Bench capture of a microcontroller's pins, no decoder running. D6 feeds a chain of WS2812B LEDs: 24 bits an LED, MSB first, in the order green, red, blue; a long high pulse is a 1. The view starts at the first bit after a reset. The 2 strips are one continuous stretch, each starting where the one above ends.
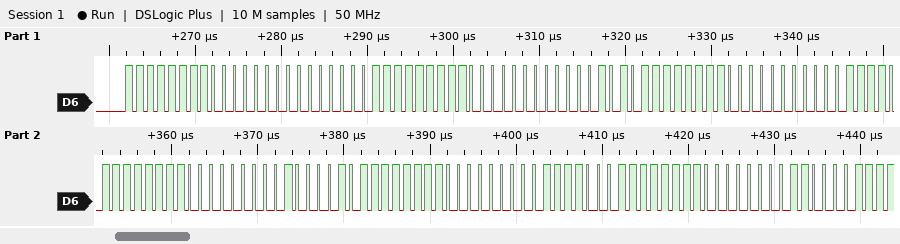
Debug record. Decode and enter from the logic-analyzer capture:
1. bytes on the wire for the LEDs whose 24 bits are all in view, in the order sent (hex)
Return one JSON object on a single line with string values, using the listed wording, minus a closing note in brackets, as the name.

{"bytes on the wire for the LEDs whose 24 bits are all in view, in the order sent": "FF 00 01 FF 00 0A FF 00 1E FF 00 42 FF 00 78 FF 00 C3"}
